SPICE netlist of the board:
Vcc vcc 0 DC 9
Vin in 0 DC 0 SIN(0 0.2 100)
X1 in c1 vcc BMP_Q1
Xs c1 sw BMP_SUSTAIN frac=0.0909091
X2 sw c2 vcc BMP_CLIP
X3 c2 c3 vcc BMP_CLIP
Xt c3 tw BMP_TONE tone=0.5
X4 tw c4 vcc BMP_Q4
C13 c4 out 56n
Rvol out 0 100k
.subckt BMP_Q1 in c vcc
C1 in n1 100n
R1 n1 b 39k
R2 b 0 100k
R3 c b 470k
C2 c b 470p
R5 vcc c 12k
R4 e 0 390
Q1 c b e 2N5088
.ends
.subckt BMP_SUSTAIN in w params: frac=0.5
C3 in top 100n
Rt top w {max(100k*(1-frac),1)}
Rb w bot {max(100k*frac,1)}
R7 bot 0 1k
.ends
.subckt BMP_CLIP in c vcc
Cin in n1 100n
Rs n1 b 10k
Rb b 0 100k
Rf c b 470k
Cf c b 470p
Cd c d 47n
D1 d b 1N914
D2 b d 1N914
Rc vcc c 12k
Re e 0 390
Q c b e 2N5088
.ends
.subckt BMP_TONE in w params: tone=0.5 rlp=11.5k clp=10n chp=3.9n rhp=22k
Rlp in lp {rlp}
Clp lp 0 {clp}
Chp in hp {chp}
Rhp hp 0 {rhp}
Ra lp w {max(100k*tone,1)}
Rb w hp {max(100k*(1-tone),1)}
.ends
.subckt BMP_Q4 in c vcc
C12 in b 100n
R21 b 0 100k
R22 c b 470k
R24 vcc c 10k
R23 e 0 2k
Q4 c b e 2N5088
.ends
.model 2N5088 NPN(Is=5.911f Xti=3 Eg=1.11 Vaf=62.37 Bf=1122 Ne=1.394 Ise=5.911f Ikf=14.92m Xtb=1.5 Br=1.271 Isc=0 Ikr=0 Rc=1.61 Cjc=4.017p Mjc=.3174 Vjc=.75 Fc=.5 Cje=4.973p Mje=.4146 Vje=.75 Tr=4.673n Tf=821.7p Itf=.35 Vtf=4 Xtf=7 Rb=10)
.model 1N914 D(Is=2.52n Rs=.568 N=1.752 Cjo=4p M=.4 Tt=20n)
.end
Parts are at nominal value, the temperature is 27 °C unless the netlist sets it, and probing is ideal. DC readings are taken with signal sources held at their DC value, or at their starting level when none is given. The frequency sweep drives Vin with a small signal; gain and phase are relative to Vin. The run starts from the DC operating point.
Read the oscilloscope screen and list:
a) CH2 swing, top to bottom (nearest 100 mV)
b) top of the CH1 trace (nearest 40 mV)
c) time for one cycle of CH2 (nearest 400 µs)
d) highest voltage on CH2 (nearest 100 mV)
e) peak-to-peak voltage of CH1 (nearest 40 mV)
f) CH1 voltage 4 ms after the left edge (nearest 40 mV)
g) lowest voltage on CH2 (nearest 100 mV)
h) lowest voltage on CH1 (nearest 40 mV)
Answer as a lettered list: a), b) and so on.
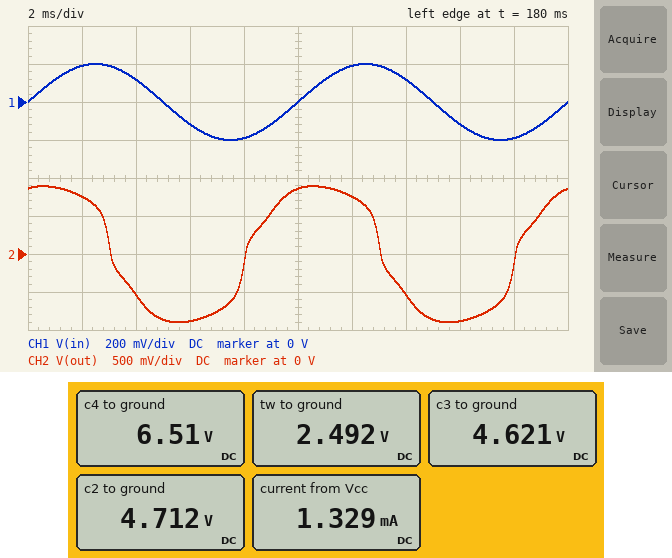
a) 1.8 V
b) 200 mV
c) 10.0 ms
d) 900 mV
e) 400 mV
f) 120 mV
g) -900 mV
h) -200 mV
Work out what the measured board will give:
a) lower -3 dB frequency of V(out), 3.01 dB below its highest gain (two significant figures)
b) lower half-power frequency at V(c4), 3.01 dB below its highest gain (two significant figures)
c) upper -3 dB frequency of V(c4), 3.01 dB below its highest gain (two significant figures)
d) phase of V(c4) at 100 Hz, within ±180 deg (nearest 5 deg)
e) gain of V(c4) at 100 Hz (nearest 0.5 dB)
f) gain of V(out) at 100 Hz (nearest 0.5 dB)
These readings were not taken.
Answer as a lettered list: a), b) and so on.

a) 76 Hz
b) 71 Hz
c) 640 Hz
d) 70 deg
e) 37.0 dB
f) 36.5 dB
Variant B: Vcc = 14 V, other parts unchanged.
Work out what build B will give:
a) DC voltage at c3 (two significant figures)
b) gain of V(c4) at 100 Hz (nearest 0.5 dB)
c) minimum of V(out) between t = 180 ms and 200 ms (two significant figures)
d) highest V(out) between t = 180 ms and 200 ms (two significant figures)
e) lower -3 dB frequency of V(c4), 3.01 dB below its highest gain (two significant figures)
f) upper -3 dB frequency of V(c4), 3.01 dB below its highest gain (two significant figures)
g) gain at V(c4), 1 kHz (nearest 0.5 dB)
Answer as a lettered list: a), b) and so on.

a) 5.7 V
b) 38.0 dB
c) -940 mV
d) 940 mV
e) 72 Hz
f) 630 Hz
g) 32.5 dB
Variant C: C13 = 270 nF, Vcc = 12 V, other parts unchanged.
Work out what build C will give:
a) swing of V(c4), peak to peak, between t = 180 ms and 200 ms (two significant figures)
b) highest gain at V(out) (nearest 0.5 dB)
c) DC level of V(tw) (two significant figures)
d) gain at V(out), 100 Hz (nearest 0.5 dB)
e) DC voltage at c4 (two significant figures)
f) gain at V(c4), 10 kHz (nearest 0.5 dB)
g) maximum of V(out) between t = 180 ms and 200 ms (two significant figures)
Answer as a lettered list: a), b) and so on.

a) 2.0 V
b) 39.0 dB
c) 2.8 V
d) 37.5 dB
e) 8.2 V
f) -7.5 dB
g) 970 mV
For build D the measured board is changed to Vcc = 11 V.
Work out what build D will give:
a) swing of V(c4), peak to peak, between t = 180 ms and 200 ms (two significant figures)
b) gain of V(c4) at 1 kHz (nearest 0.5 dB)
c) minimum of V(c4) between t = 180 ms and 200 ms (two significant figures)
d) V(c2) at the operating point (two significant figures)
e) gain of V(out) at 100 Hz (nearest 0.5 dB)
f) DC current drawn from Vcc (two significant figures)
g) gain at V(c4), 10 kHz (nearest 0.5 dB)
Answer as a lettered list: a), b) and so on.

a) 2.0 V
b) 32.0 dB
c) 6.6 V
d) 5.1 V
e) 37.0 dB
f) 1.8 mA
g) -7.5 dB
